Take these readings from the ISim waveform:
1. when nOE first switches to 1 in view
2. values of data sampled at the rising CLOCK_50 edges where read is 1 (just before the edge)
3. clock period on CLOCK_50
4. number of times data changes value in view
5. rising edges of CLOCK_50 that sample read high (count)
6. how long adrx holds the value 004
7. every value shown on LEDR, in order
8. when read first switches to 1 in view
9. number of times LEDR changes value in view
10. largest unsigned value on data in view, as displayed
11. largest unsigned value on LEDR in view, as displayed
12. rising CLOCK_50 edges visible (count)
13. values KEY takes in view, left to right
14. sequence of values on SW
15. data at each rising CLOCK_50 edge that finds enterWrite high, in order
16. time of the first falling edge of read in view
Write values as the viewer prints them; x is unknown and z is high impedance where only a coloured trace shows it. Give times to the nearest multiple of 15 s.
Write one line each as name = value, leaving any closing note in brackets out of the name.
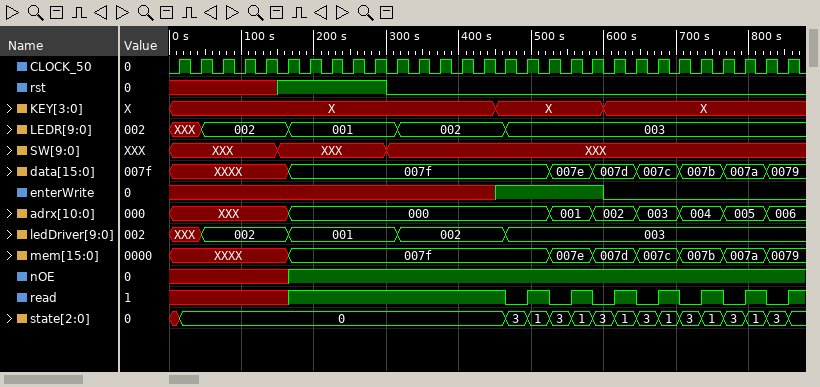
when nOE first switches to 1 in view = 165 s
values of data sampled at the rising CLOCK_50 edges where read is 1 = 007f, 007f, 007f, 007f, 007f, 007f, 007f, 007f, 007f, 007f, 007f, 007e, 007d, 007c, 007b, 007a
clock period on CLOCK_50 = 30 s
number of times data changes value in view = 7
rising edges of CLOCK_50 that sample read high = 16
how long adrx holds the value 004 = 60 s
every value shown on LEDR, in order = XXX, 002, 001, 002, 003
when read first switches to 1 in view = 165 s
number of times LEDR changes value in view = 4
largest unsigned value on data in view, as displayed = 007f
largest unsigned value on LEDR in view, as displayed = 003
rising CLOCK_50 edges visible = 29
values KEY takes in view, left to right = X, X, X
sequence of values on SW = XXX, XXX, XXX
data at each rising CLOCK_50 edge that finds enterWrite high, in order = 007f, 007f, 007f, 007e, 007e
time of the first falling edge of read in view = 465 s
